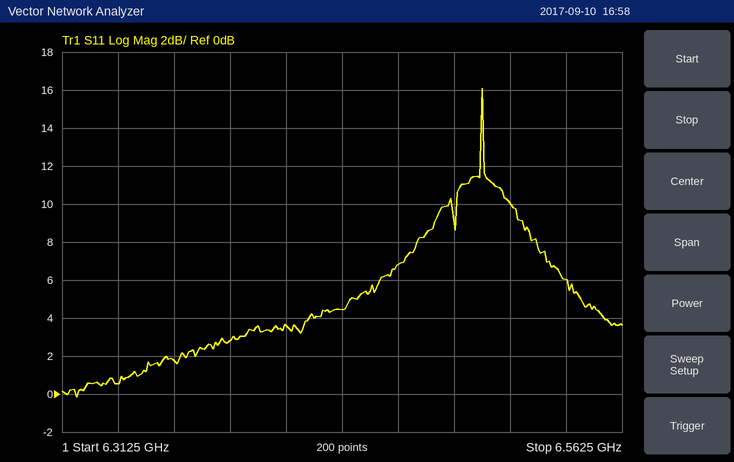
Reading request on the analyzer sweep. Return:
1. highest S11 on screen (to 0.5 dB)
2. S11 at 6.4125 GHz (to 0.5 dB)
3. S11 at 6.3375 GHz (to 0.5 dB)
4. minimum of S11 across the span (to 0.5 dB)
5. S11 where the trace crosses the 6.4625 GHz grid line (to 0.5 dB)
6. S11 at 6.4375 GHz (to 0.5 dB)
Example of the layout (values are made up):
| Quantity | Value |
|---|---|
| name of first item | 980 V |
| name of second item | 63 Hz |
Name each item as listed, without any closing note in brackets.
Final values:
| Quantity | Value |
|---|---|
| highest S11 on screen | 16.0 dB |
| S11 at 6.4125 GHz | 3.5 dB |
| S11 at 6.3375 GHz | 0.5 dB |
| minimum of S11 across the span | 0.0 dB |
| S11 where the trace crosses the 6.4625 GHz grid line | 7.0 dB |
| S11 at 6.4375 GHz | 4.5 dB |
